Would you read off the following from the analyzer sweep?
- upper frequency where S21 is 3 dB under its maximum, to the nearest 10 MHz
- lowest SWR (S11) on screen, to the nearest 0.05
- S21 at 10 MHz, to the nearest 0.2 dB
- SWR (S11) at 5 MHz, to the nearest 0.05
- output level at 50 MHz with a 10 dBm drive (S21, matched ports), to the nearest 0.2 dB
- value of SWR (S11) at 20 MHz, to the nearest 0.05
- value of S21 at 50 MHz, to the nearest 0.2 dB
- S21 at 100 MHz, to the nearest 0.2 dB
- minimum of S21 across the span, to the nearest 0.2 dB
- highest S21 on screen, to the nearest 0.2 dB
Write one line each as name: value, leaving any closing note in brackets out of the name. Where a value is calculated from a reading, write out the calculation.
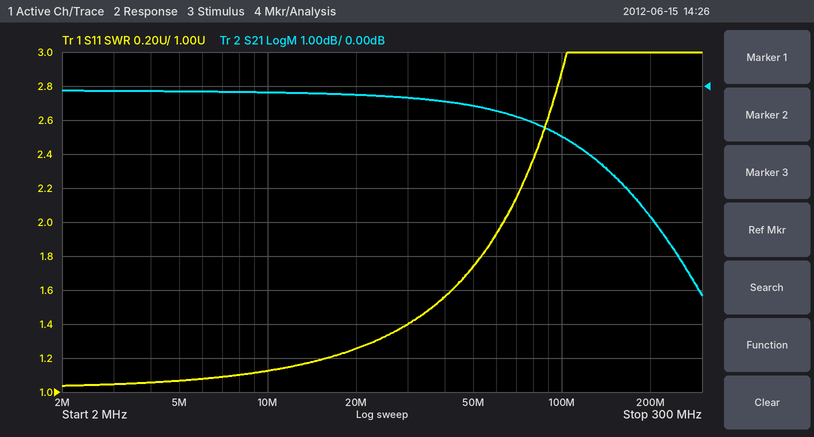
upper frequency where S21 is 3 dB under its maximum, to the nearest 10 MHz: 170 MHz
lowest SWR (S11) on screen, to the nearest 0.05: 1.05
S21 at 10 MHz, to the nearest 0.2 dB: -0.2 dB
SWR (S11) at 5 MHz, to the nearest 0.05: 1.05
output level at 50 MHz with a 10 dBm drive (S21, matched ports), to the nearest 0.2 dB: 10 dBm + (-0.6 dB) = 9.4 dBm
value of SWR (S11) at 20 MHz, to the nearest 0.05: 1.25
value of S21 at 50 MHz, to the nearest 0.2 dB: -0.6 dB
S21 at 100 MHz, to the nearest 0.2 dB: -1.4 dB
minimum of S21 across the span, to the nearest 0.2 dB: -6.2 dB
highest S21 on screen, to the nearest 0.2 dB: -0.2 dB
